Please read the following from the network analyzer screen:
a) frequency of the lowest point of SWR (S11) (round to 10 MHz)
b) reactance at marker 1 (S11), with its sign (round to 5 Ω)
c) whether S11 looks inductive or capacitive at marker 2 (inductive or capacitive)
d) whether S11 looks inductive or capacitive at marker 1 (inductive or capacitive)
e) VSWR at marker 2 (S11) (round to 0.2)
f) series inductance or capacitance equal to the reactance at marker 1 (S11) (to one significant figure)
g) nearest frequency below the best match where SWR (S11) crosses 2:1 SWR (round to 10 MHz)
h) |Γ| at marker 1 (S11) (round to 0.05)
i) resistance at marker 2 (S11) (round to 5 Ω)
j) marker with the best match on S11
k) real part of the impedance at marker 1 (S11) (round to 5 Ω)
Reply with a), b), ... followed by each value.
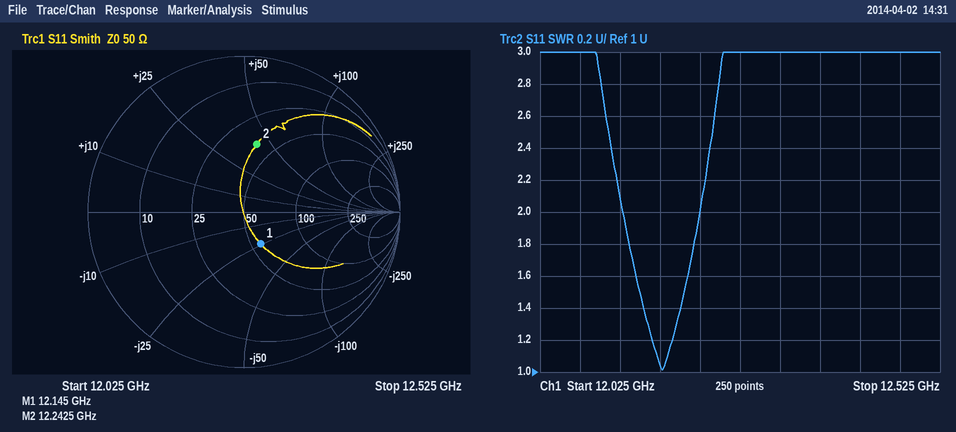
a) 12.18 GHz
b) -25 Ω
c) inductive
d) capacitive
e) 2.6
f) 500 fF
g) 12.13 GHz
h) 0.25
i) 40 Ω
j) marker 1
k) 55 Ω
